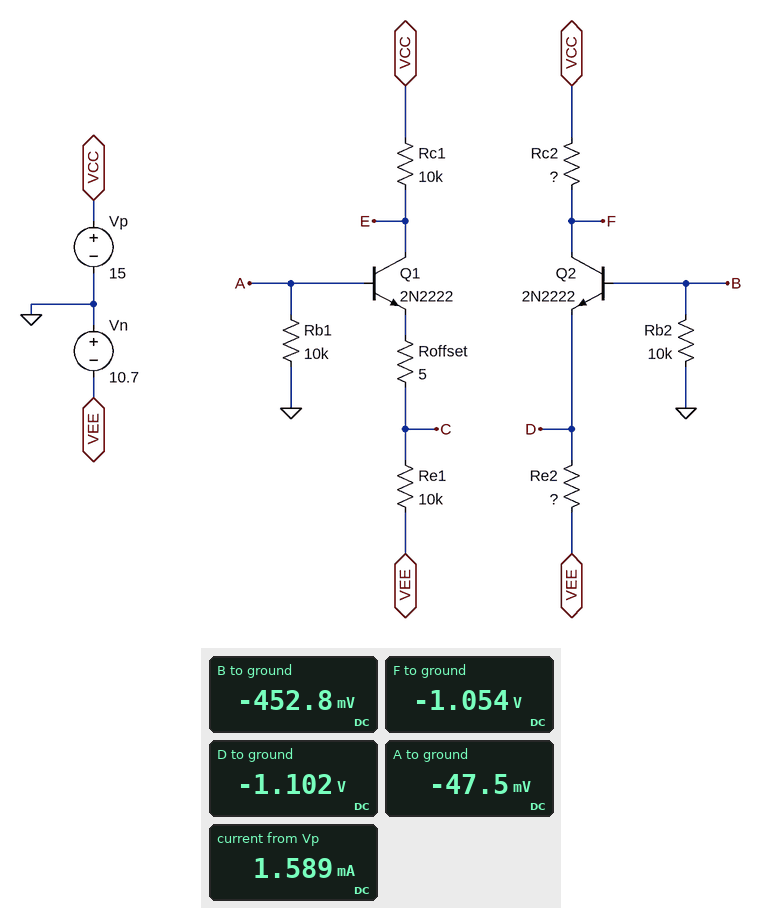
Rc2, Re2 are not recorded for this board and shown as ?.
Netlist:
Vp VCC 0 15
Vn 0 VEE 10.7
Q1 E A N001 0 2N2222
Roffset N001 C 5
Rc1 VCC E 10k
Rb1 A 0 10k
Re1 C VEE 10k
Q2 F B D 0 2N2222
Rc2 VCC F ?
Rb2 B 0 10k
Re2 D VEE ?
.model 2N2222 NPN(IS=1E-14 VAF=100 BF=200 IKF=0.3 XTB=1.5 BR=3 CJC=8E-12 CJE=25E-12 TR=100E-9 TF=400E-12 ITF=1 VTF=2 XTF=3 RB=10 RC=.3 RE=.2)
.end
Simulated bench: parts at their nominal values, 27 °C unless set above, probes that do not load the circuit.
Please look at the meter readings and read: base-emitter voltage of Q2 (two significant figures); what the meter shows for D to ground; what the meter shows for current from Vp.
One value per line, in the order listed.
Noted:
650 mV
-1.102 V
1.589 mA
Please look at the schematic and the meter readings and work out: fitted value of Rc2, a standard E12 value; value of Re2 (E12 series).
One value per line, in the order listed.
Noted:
27 kΩ
15 kΩ
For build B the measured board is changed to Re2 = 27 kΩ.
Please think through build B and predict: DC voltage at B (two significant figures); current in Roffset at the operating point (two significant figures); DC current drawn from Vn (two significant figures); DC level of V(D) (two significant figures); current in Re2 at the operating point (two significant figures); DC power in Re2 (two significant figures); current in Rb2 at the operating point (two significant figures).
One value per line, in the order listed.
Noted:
-18 mV
1.0 mA
1.4 mA
-650 mV
370 µA
3.7 mW
1.8 µA
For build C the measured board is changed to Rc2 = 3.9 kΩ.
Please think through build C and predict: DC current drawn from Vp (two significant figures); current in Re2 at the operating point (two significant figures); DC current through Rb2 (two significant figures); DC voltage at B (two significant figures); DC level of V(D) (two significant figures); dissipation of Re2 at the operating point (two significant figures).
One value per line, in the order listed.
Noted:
1.7 mA
670 µA
3.0 µA
-30 mV
-670 mV
6.7 mW
